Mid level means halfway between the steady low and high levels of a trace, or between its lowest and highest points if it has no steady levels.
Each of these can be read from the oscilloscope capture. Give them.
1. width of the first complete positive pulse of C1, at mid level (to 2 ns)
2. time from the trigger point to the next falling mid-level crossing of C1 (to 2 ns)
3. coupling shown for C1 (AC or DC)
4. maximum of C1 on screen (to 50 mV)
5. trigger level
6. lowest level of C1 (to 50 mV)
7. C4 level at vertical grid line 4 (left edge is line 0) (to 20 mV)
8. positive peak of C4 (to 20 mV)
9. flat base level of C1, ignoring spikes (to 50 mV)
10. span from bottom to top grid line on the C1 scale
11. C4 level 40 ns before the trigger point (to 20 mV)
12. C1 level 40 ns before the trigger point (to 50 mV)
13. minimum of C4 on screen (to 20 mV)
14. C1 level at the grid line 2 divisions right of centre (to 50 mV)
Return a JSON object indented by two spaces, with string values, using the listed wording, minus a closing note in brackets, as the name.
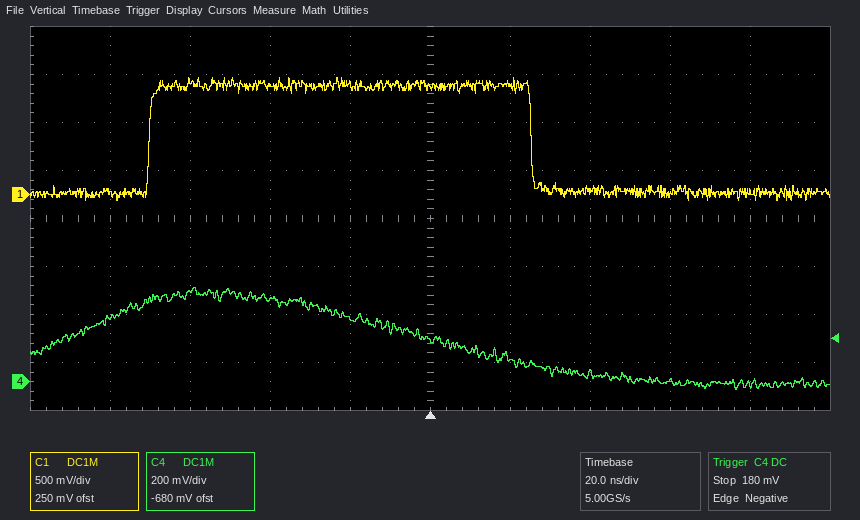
{
  "width of the first complete positive pulse of C1, at mid level": "96 ns",
  "time from the trigger point to the next falling mid-level crossing of C1": "26 ns",
  "coupling shown for C1": "DC",
  "maximum of C1 on screen": "1.20 V",
  "trigger level": "180 mV",
  "lowest level of C1": "-50 mV",
  "C4 level at vertical grid line 4 (left edge is line 0)": "260 mV",
  "positive peak of C4": "400 mV",
  "flat base level of C1, ignoring spikes": "0 mV",
  "span from bottom to top grid line on the C1 scale": "4 V",
  "C4 level 40 ns before the trigger point": "340 mV",
  "C1 level 40 ns before the trigger point": "1.10 V",
  "minimum of C4 on screen": "-40 mV",
  "C1 level at the grid line 2 divisions right of centre": "50 mV"
}
